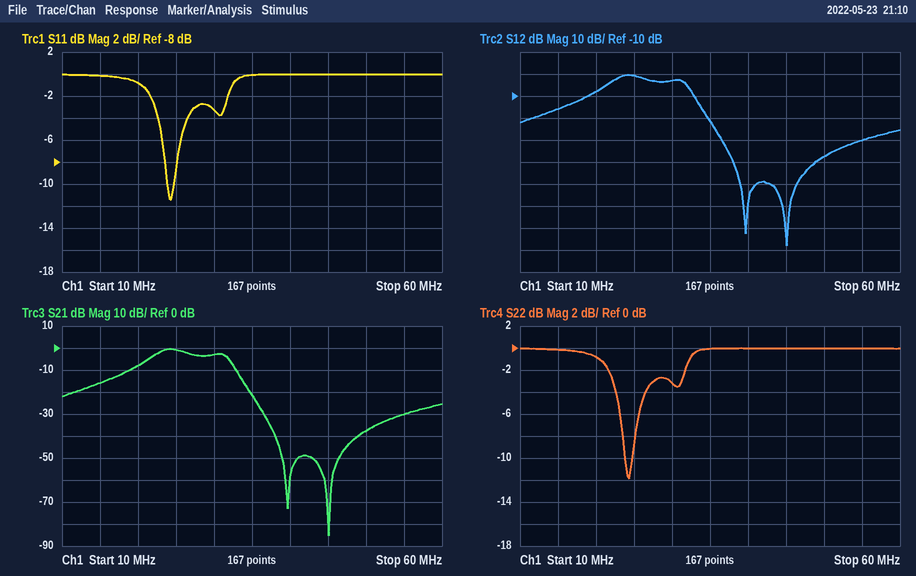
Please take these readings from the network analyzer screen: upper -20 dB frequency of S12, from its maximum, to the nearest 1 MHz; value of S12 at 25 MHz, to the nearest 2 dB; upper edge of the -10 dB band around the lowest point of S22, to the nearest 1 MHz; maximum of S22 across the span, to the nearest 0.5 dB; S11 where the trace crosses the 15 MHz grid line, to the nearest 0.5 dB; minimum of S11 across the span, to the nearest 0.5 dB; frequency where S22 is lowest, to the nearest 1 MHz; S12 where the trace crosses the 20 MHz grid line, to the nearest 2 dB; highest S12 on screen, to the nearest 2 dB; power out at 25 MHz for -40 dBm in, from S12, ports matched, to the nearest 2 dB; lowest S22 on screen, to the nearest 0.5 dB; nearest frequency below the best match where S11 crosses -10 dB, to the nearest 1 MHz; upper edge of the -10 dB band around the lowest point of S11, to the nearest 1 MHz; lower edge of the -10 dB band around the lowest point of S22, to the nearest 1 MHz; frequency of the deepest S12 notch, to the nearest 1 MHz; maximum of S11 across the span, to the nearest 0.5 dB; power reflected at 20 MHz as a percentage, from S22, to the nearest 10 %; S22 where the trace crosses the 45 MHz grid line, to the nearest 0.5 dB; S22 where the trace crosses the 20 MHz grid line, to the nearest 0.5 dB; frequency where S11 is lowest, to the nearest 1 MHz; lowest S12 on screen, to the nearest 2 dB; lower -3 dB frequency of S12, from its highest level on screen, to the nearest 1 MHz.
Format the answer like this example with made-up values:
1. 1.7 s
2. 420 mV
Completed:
1. 35 MHz
2. 0 dB
3. 25 MHz
4. 0.0 dB
5. 0.0 dB
6. -11.5 dB
7. 24 MHz
8. -8 dB
9. 0 dB
10. -40 dBm
11. -12.0 dB
12. 24 MHz
13. 25 MHz
14. 24 MHz
15. 45 MHz
16. 0.0 dB
17. 80 %
18. 0.0 dB
19. -1.0 dB
20. 24 MHz
21. -78 dB
22. 22 MHz
